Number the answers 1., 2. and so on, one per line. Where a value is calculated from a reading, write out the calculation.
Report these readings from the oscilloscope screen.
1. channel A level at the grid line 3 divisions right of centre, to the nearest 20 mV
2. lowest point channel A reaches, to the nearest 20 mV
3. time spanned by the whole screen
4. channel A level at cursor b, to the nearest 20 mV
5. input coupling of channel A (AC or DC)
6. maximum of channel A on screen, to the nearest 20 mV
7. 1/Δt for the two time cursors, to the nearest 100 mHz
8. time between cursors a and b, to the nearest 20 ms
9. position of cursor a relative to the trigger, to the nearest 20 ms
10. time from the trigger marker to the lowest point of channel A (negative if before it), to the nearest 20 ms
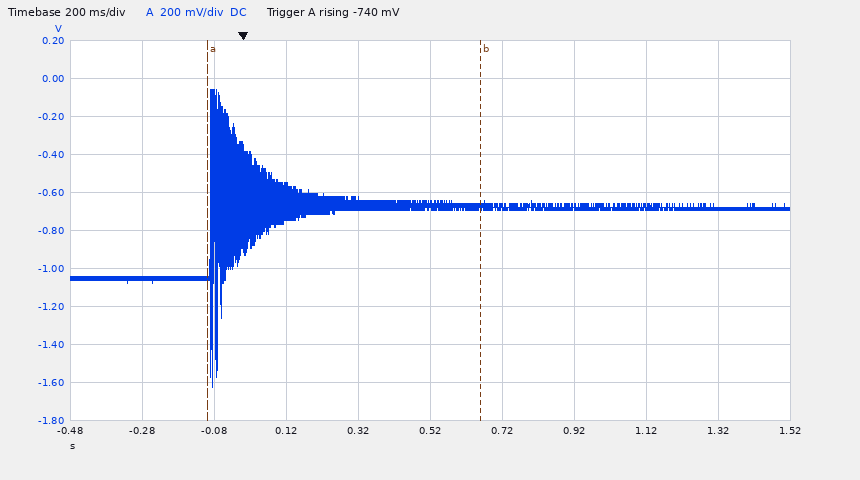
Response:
1. -680 mV
2. -1.62 V
3. 2 s
4. -680 mV
5. DC
6. -60 mV
7. 1 / 760 ms ≈ 1.3 Hz
8. 760 ms
9. -100 ms
10. -80 ms
